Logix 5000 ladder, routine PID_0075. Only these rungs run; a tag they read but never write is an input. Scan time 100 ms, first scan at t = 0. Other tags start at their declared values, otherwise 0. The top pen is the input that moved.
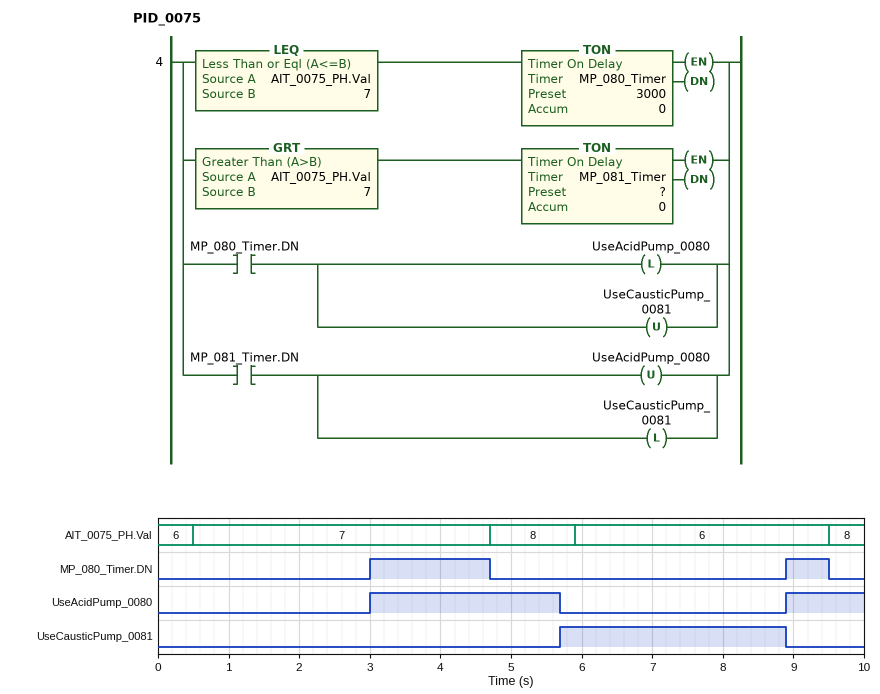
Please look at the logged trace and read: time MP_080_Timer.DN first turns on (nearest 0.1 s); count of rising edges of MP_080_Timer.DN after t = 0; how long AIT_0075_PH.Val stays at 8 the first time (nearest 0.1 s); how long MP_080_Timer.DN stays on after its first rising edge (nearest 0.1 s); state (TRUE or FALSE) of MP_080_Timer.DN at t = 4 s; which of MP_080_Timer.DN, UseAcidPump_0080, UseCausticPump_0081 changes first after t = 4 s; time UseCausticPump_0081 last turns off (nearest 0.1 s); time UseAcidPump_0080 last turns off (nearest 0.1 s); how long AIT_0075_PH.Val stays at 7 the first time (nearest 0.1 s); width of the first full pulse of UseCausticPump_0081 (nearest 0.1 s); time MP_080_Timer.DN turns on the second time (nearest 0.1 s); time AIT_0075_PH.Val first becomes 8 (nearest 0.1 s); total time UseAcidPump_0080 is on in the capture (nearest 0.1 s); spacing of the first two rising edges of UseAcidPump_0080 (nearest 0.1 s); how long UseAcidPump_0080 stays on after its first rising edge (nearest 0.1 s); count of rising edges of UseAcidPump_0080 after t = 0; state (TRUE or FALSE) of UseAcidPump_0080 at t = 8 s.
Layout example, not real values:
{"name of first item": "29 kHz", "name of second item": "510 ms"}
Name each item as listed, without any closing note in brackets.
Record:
{"time MP_080_Timer.DN first turns on": "3.0 s", "count of rising edges of MP_080_Timer.DN after t = 0": "2", "how long AIT_0075_PH.Val stays at 8 the first time": "1.2 s", "how long MP_080_Timer.DN stays on after its first rising edge": "1.7 s", "state (TRUE or FALSE) of MP_080_Timer.DN at t = 4 s": "TRUE", "which of MP_080_Timer.DN, UseAcidPump_0080, UseCausticPump_0081 changes first after t = 4 s": "MP_080_Timer.DN", "time UseCausticPump_0081 last turns off": "8.9 s", "time UseAcidPump_0080 last turns off": "5.7 s", "how long AIT_0075_PH.Val stays at 7 the first time": "4.2 s", "width of the first full pulse of UseCausticPump_0081": "3.2 s", "time MP_080_Timer.DN turns on the second time": "8.9 s", "time AIT_0075_PH.Val first becomes 8": "4.7 s", "total time UseAcidPump_0080 is on in the capture": "3.8 s", "spacing of the first two rising edges of UseAcidPump_0080": "5.9 s", "how long UseAcidPump_0080 stays on after its first rising edge": "2.7 s", "count of rising edges of UseAcidPump_0080 after t = 0": "2", "state (TRUE or FALSE) of UseAcidPump_0080 at t = 8 s": "FALSE"}
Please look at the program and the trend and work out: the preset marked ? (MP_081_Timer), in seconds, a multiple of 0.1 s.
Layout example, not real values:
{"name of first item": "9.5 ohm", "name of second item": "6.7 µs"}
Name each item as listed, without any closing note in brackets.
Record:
{"the preset marked ? (MP_081_Timer), in seconds, a multiple of 0.1 s": "1.0 s"}
